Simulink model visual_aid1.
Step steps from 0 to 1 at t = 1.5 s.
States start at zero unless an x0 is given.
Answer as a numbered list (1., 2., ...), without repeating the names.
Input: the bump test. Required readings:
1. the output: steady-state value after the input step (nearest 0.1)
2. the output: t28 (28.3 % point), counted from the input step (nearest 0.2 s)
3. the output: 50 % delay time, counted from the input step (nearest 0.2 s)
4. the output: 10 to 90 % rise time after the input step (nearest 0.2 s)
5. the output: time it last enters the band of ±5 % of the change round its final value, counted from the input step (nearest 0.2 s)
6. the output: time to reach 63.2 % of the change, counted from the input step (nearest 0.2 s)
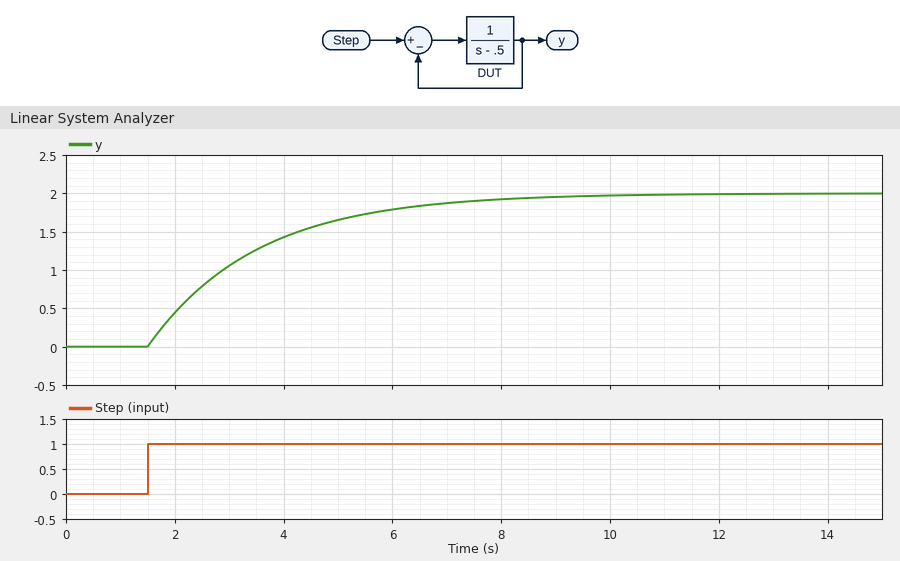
1. 2.0
2. 0.6 s
3. 1.4 s
4. 4.4 s
5. 6.0 s
6. 2.0 s
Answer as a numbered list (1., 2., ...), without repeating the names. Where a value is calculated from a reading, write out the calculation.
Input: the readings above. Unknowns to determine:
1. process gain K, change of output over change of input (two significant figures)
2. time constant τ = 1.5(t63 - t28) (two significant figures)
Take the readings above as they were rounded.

1. (2 - 0) / 1 = 2.0
2. 1.5 × (2 - 0.6) = 2.1 s
